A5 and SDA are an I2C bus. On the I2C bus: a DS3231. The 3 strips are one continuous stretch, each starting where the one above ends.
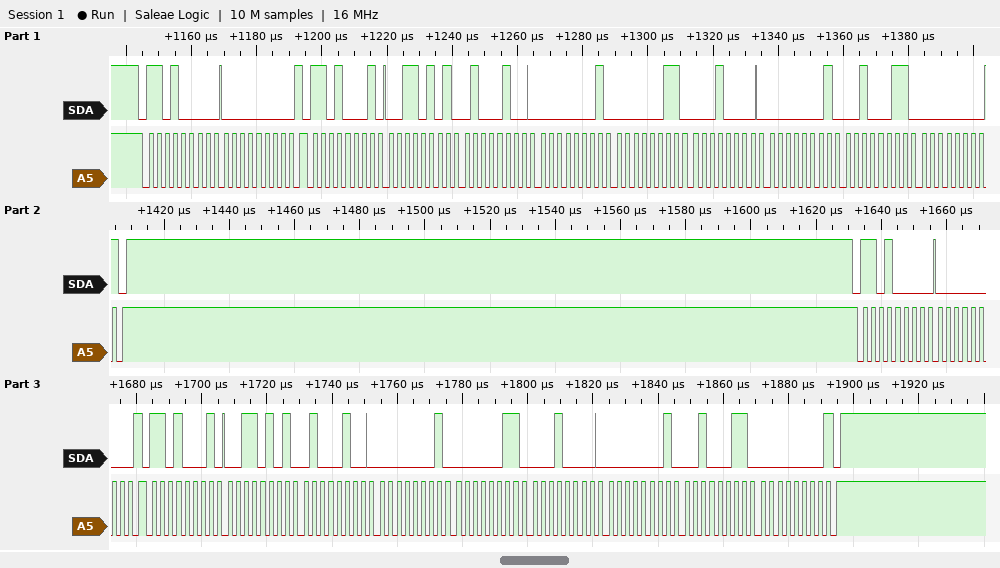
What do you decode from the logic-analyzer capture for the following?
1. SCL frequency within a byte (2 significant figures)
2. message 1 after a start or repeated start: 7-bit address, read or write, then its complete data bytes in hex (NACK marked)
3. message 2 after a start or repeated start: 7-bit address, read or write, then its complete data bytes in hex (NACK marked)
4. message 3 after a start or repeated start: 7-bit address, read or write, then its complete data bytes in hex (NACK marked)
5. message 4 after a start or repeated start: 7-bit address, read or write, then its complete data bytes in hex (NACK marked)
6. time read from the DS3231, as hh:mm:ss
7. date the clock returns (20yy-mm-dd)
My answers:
400 kHz
0x68 write: 00
0x68 read: 35 44 01 03 10 01 23 00 NACK
0x68 write: 00
0x68 read: 35 44 01 03 10 01 23 00 NACK
01:44:35
2023-01-10
